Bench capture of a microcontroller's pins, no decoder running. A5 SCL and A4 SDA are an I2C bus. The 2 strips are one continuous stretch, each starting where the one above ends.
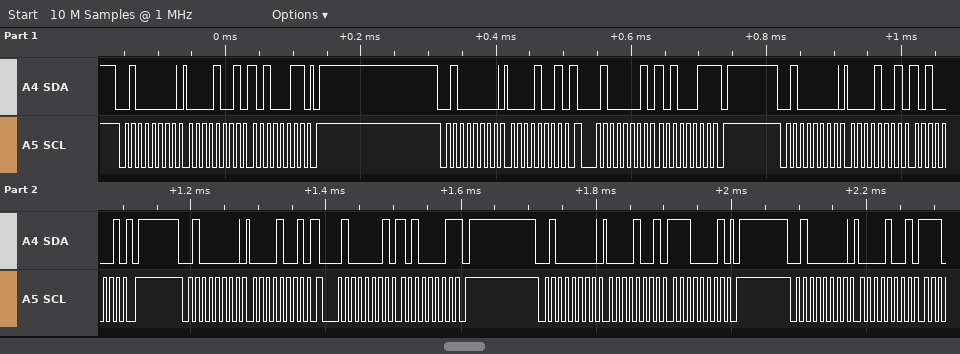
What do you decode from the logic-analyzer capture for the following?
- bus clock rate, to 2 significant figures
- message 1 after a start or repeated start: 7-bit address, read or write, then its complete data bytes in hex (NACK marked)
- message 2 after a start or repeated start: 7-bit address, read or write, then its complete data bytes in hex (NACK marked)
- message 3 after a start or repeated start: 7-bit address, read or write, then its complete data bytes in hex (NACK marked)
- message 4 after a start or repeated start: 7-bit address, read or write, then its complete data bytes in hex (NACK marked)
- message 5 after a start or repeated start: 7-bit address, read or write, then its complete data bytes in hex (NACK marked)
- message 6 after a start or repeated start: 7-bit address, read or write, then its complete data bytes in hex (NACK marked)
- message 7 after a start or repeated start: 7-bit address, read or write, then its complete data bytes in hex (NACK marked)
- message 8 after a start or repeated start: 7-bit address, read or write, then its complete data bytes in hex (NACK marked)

100 kHz
0x20 write: 09 A3
0x20 write: 09
0x20 read: A3 NACK
0x20 write: 09 A1
0x20 write: 09
0x20 read: A1 NACK
0x20 write: 09 E1
0x20 write: 09
